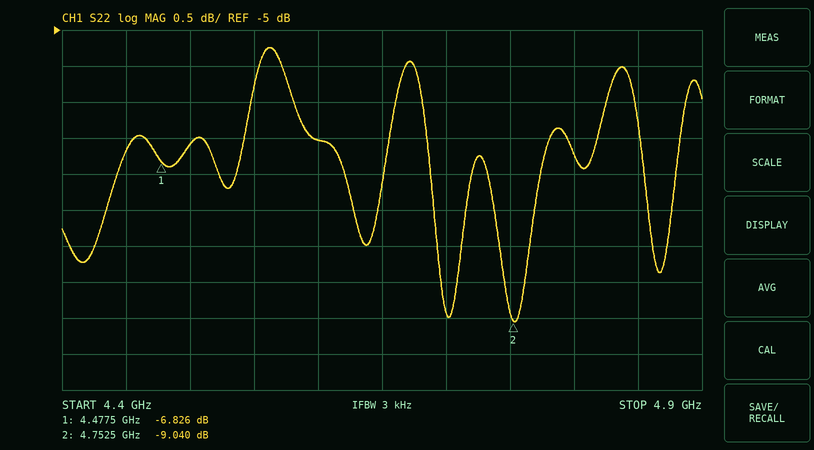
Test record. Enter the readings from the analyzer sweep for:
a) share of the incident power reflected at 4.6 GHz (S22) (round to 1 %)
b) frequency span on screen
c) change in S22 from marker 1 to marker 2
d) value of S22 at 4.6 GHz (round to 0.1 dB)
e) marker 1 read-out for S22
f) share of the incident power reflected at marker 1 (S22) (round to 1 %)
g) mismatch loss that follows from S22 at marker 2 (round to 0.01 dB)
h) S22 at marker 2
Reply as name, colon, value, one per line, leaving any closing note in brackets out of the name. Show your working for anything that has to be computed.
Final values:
share of the incident power reflected at 4.6 GHz (S22): 10^(-6.5/10) ≈ 22 %
frequency span on screen: 500 MHz
change in S22 from marker 1 to marker 2: -9.04 − (-6.826) = -2.214 dB
value of S22 at 4.6 GHz: -6.5 dB
marker 1 read-out for S22: -6.826 dB
share of the incident power reflected at marker 1 (S22): 10^(-6.826/10) ≈ 21 %
mismatch loss that follows from S22 at marker 2: −10 log10(1 − 10^(-9.04/10)) ≈ 0.58 dB
S22 at marker 2: -9.040 dB
